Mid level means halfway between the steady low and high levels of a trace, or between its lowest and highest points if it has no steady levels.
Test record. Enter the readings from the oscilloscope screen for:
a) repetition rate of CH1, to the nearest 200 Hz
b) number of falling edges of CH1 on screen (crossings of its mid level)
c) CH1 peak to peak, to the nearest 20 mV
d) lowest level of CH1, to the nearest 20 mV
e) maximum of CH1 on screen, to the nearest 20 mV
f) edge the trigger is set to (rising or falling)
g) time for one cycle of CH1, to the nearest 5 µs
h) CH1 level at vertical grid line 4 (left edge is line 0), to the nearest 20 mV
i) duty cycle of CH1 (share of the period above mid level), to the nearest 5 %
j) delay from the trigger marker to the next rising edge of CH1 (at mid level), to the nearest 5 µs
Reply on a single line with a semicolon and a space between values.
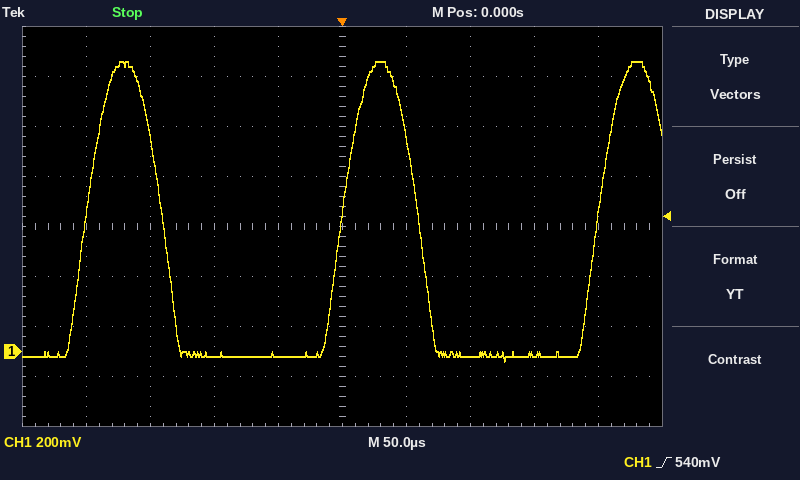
5.0 kHz; 2; 1.20 V; -40 mV; 1.16 V; rising; 200 µs; -20 mV; 30 %; 200 µs
